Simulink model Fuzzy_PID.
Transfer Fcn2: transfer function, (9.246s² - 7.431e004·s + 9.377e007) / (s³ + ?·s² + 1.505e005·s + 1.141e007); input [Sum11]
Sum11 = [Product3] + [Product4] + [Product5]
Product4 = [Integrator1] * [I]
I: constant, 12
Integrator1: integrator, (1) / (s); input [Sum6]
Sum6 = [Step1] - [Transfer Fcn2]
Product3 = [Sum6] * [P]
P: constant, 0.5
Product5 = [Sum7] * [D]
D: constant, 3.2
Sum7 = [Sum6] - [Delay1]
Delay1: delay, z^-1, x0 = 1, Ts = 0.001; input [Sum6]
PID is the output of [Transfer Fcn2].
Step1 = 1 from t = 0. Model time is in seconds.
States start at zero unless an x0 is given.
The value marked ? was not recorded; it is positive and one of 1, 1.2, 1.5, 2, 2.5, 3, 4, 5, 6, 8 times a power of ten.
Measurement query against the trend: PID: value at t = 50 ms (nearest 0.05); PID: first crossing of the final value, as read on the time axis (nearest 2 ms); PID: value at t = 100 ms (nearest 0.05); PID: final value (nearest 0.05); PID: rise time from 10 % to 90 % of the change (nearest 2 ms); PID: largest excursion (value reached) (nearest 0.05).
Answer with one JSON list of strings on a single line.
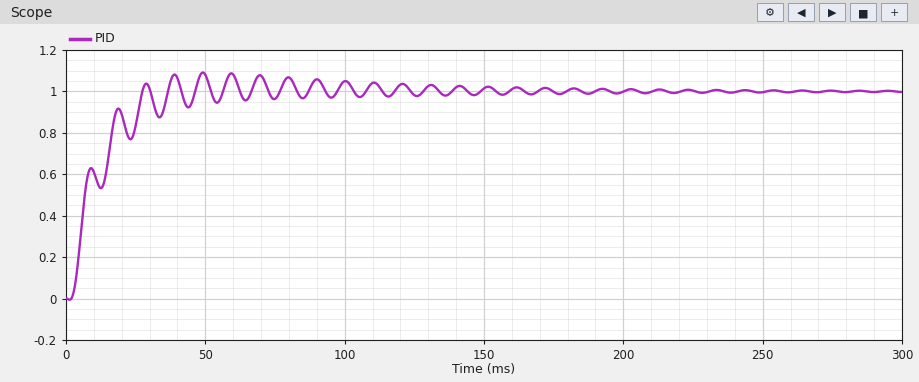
["1.10", "28 ms", "1.05", "1.00", "14 ms", "1.10"]
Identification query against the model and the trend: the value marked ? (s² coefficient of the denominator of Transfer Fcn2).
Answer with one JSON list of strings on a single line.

["800"]
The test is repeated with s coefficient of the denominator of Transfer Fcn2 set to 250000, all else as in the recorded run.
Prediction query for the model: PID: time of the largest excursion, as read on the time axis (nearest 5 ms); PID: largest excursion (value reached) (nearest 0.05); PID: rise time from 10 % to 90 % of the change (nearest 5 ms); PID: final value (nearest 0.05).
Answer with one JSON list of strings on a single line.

["55 ms", "1.05", "20 ms", "1.00"]
